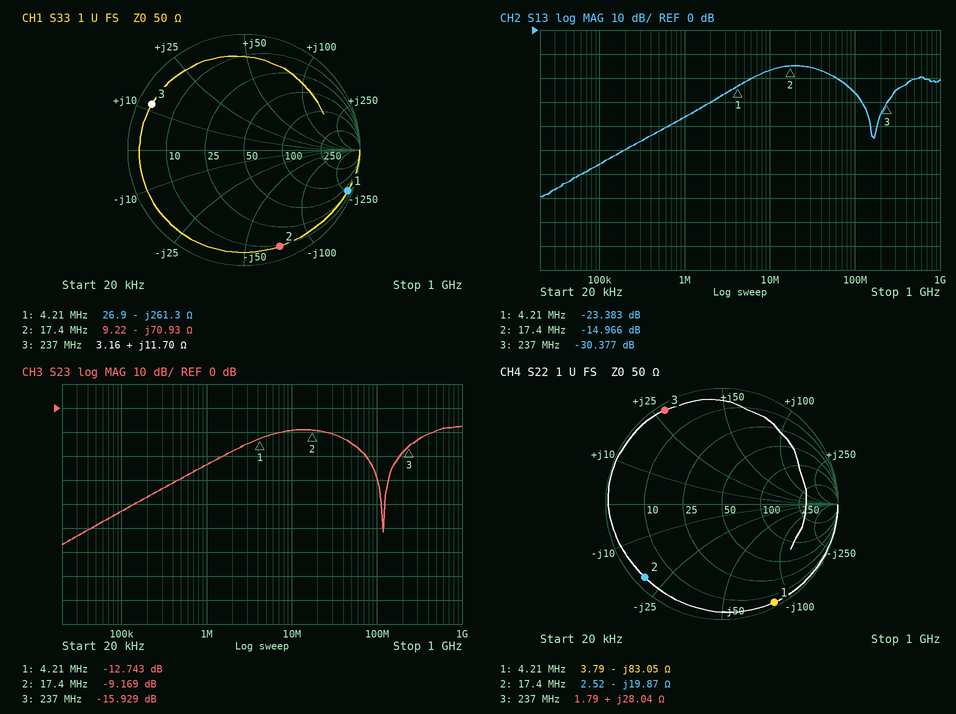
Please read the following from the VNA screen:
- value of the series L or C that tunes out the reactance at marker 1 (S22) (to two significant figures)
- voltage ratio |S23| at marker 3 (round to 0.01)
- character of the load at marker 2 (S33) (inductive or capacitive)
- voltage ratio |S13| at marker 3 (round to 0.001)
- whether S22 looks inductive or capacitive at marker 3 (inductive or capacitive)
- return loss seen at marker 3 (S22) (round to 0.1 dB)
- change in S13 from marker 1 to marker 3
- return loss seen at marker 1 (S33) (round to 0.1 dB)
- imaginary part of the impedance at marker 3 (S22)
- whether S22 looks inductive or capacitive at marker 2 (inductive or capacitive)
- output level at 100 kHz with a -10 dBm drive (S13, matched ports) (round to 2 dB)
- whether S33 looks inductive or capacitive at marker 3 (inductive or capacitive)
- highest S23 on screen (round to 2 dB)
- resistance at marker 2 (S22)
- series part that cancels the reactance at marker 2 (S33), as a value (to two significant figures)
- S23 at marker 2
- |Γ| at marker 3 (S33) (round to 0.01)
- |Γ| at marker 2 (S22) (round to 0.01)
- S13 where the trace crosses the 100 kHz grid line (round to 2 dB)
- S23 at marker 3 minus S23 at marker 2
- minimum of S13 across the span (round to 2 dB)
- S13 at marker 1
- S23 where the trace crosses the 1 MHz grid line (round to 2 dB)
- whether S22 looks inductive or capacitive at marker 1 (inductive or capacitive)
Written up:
3.1 µH
0.16
capacitive
0.030
inductive
0.5 dB
-6.994 dB
0.3 dB
+28.04 Ω
capacitive
-66 dBm
inductive
-8 dB
2.52 Ω
650 nH
-9.169 dB
0.89
0.92
-56 dB
-6.760 dB
-70 dB
-23.383 dB
-24 dB
capacitive
